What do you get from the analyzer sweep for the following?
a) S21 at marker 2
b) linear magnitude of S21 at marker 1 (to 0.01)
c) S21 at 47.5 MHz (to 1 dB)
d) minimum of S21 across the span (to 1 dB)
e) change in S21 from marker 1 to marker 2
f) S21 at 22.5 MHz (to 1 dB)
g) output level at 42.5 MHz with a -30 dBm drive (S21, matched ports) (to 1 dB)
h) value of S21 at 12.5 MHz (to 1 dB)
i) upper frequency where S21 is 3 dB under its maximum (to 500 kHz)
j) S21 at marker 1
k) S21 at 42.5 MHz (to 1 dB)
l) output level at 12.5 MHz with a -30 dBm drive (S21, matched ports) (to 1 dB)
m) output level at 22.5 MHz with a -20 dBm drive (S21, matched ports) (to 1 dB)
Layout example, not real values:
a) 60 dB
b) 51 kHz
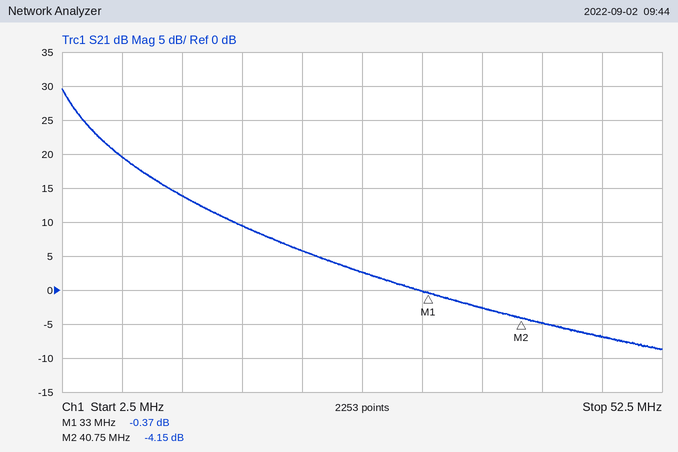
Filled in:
a) -4.15 dB
b) 0.96
c) -7 dB
d) -9 dB
e) -3.78 dB
f) 6 dB
g) -35 dBm
h) 14 dB
i) 3.5 MHz
j) -0.37 dB
k) -5 dB
l) -16 dBm
m) -14 dBm
